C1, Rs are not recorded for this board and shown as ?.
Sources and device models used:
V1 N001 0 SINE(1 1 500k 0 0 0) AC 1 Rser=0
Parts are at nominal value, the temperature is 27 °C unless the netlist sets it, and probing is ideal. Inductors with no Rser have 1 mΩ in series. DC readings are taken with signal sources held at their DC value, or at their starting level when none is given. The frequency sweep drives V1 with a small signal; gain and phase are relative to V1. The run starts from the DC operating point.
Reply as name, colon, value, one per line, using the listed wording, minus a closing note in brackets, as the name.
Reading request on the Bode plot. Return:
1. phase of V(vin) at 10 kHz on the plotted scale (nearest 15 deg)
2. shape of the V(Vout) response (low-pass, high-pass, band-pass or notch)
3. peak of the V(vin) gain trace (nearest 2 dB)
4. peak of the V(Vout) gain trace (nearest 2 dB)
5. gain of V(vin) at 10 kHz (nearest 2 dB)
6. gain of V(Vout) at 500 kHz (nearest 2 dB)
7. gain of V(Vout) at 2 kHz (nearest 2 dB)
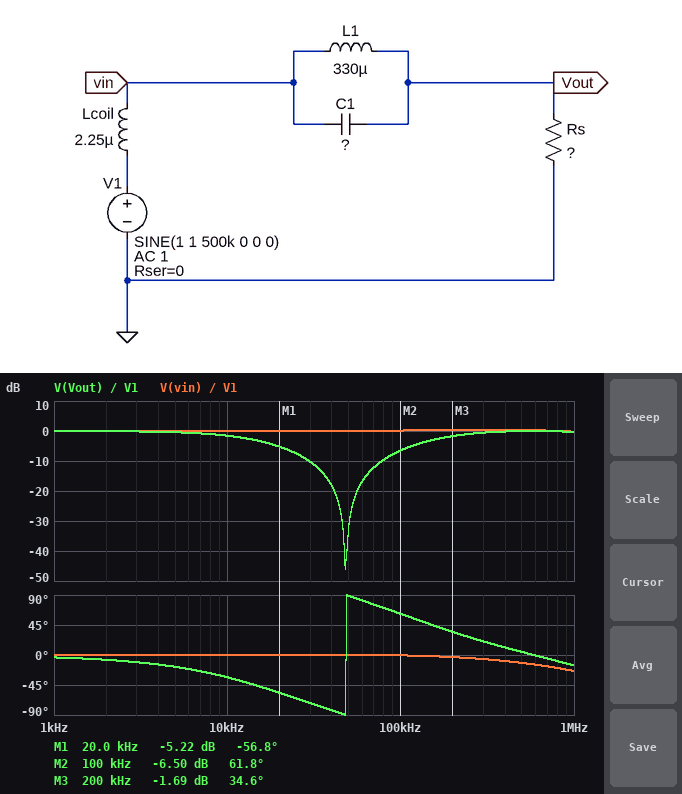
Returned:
phase of V(vin) at 10 kHz on the plotted scale: 0 deg
shape of the V(Vout) response: notch
peak of the V(vin) gain trace: 0 dB
peak of the V(Vout) gain trace: 0 dB
gain of V(vin) at 10 kHz: 0 dB
gain of V(Vout) at 500 kHz: 0 dB
gain of V(Vout) at 2 kHz: 0 dB
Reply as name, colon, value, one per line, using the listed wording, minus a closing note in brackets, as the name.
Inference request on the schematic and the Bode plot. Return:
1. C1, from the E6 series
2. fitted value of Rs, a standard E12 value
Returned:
C1, from the E6 series: 33 nF
fitted value of Rs, a standard E12 value: 33 Ω
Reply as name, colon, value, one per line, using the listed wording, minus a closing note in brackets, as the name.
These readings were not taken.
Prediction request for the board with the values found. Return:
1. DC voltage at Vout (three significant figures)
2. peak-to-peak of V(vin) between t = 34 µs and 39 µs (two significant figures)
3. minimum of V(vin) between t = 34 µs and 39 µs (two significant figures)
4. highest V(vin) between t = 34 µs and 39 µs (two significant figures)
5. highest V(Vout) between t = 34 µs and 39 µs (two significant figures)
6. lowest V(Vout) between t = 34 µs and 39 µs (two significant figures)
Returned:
DC voltage at Vout: 1.00 V
peak-to-peak of V(vin) between t = 34 µs and 39 µs: 2.1 V
minimum of V(vin) between t = 34 µs and 39 µs: -39 mV
highest V(vin) between t = 34 µs and 39 µs: 2.0 V
highest V(Vout) between t = 34 µs and 39 µs: 2.0 V
lowest V(Vout) between t = 34 µs and 39 µs: 3.9 mV
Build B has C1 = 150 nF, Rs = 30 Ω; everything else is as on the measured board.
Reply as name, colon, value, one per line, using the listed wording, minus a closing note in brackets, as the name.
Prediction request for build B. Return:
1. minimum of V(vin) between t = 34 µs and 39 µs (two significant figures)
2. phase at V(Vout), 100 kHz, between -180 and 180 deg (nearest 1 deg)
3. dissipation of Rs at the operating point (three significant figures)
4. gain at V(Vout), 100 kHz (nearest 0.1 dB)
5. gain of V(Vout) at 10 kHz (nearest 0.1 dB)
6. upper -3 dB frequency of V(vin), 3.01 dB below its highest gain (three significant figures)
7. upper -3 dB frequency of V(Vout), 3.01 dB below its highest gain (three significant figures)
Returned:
minimum of V(vin) between t = 34 µs and 39 µs: 11 mV
phase at V(Vout), 100 kHz, between -180 and 180 deg: 18 deg
dissipation of Rs at the operating point: 33.3 mW
gain at V(Vout), 100 kHz: -0.4 dB
gain of V(Vout) at 10 kHz: -2.4 dB
upper -3 dB frequency of V(vin), 3.01 dB below its highest gain: 2.10 MHz
upper -3 dB frequency of V(Vout), 3.01 dB below its highest gain: 2.16 MHz
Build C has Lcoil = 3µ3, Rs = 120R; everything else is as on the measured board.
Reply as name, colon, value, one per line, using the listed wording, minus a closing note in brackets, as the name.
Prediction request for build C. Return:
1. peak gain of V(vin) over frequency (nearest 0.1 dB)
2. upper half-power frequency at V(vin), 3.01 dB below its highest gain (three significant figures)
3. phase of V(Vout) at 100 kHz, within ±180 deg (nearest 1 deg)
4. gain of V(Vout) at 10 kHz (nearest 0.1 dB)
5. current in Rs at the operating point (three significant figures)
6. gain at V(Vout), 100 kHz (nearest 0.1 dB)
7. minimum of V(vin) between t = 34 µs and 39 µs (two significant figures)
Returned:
peak gain of V(vin) over frequency: 0.1 dB
upper half-power frequency at V(vin), 3.01 dB below its highest gain: 5.75 MHz
phase of V(Vout) at 100 kHz, within ±180 deg: 27 deg
gain of V(Vout) at 10 kHz: -0.1 dB
current in Rs at the operating point: 8.33 mA
gain at V(Vout), 100 kHz: -1.0 dB
minimum of V(vin) between t = 34 µs and 39 µs: -3.3 mV
